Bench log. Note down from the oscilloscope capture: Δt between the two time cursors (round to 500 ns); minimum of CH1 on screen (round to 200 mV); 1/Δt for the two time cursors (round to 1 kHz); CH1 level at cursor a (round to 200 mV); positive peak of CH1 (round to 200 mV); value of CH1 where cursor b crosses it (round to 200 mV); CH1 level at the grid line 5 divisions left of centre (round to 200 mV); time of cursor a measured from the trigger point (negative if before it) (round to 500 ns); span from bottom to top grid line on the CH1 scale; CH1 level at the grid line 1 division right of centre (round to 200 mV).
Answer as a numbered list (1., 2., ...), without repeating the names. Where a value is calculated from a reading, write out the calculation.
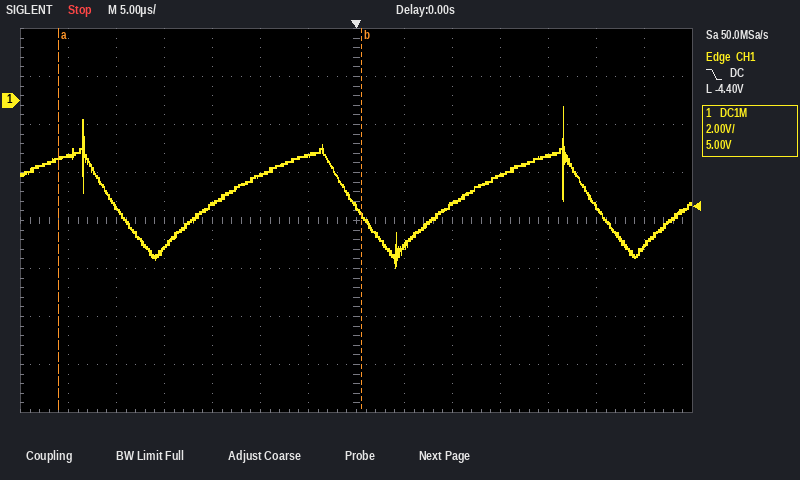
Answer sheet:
1. 31.5 µs
2. -7.0 V
3. 1 / 31.5 µs ≈ 32 kHz
4. -2.4 V
5. -200 mV
6. -4.8 V
7. -4.4 V
8. -31.0 µs
9. 16 V
10. -6.0 V
